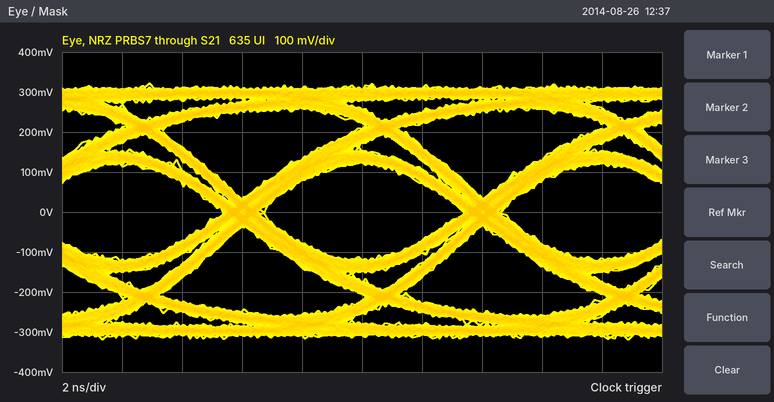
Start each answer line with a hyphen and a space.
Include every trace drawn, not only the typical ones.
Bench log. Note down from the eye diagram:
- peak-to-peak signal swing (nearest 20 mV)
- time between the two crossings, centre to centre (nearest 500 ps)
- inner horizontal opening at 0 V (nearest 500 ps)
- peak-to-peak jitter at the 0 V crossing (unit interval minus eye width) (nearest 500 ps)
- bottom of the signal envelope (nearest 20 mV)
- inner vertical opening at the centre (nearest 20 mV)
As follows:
- 640 mV
- 8.0 ns
- 6.5 ns
- 1.5 ns
- -320 mV
- 240 mV
